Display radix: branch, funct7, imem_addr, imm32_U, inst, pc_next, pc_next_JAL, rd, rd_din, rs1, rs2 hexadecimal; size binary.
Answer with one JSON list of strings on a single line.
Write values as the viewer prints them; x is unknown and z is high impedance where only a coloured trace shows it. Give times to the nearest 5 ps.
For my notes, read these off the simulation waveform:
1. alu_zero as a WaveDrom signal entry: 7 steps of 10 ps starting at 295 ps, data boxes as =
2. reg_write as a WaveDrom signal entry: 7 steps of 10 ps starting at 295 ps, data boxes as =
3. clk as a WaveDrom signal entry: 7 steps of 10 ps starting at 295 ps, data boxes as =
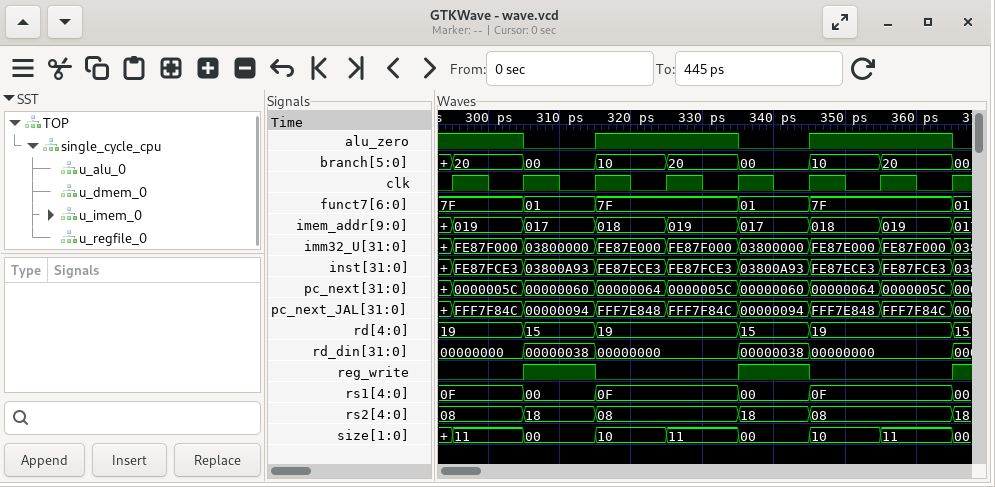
["{name: 'alu_zero', wave: '101.01.'}", "{name: 'reg_write', wave: '010.10.'}", "{name: 'clk', wave: 'p......'}"]
